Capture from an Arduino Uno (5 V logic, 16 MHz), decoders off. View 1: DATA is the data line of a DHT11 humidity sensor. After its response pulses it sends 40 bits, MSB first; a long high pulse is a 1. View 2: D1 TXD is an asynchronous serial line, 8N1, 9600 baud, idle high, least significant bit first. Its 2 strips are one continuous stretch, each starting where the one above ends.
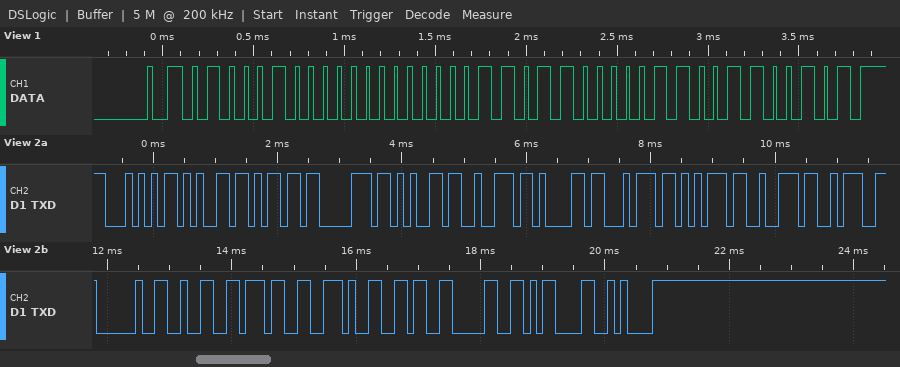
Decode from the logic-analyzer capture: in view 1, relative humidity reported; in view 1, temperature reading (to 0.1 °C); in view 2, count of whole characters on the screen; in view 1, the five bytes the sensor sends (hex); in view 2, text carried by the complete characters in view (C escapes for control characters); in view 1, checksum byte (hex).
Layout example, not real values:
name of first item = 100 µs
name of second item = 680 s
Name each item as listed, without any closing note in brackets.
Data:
in view 1, relative humidity reported = 68 %
in view 1, temperature reading = 27.6 °C
in view 2, count of whole characters on the screen = 19
in view 1, the five bytes the sensor sends = 44 00 1B 06 65
in view 2, text carried by the complete characters in view = "Temperatur: 27.60\r\n"
in view 1, checksum byte = 0x65
